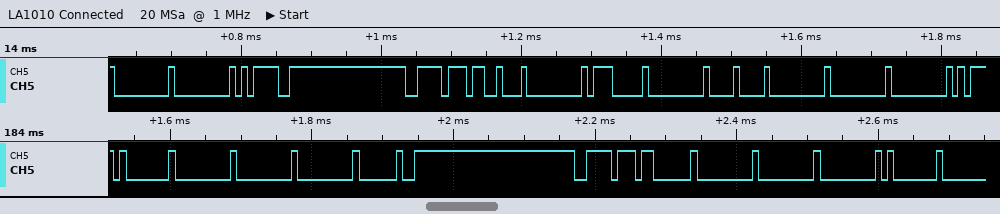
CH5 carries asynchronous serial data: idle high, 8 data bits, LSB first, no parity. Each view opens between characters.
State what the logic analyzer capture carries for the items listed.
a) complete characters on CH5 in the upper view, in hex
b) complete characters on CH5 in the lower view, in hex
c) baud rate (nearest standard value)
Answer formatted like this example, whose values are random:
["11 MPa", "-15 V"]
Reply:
["00, 00, 3D, DE, 13, 00, 07, 00, 08, 00, 00, 00", "01, 00, 00, 00, 20, DE, 03, 00, 00, 00, 01", "115200 baud"]
